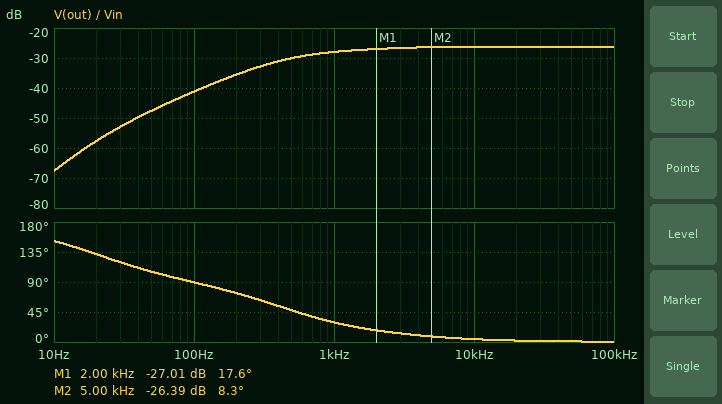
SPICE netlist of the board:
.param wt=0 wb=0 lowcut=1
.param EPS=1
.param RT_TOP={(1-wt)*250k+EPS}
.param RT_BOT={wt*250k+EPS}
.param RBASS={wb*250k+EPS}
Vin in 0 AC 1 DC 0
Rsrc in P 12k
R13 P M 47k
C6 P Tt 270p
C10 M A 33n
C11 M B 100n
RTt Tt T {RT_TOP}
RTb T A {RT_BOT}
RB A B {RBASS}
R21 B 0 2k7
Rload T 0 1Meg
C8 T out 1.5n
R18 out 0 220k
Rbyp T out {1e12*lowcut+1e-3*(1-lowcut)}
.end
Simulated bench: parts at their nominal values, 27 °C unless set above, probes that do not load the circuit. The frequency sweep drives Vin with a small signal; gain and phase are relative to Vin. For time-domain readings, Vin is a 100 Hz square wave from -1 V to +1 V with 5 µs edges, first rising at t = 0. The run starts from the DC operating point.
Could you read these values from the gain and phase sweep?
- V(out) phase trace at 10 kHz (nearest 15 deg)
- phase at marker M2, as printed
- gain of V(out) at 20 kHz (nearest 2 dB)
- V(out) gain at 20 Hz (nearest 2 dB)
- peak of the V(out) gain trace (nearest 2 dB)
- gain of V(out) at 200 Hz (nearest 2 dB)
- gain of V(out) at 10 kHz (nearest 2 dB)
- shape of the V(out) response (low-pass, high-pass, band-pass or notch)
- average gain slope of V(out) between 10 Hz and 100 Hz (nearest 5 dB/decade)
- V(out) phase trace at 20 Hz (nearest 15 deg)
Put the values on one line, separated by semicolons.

0 deg; 8.3 deg; -26 dB; -58 dB; -26 dB; -36 dB; -26 dB; high-pass; 25 dB/decade; 135 deg
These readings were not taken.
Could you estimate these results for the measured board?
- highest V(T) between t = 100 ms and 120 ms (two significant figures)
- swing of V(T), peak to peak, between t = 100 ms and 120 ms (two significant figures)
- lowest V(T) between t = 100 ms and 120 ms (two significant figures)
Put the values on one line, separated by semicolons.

67 mV; 130 mV; -67 mV
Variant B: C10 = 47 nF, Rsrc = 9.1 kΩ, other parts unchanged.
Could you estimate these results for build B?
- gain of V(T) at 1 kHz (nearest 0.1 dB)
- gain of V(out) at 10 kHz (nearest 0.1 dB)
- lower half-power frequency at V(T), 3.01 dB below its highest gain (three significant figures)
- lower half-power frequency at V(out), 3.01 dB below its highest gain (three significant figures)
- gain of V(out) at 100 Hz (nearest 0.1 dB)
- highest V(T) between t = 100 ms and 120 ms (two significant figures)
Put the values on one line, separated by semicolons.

-26.6 dB; -25.8 dB; 24.5 Hz; 635 Hz; -40.8 dB; 70 mV
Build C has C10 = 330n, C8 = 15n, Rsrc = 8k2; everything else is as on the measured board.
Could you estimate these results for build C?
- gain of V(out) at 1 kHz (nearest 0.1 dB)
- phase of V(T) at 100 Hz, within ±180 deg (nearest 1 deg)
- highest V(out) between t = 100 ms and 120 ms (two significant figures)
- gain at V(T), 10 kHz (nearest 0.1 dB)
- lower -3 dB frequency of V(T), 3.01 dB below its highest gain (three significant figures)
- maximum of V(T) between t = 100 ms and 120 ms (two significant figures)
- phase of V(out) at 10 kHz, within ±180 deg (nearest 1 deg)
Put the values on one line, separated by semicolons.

-26.5 dB; 4 deg; 92 mV; -25.6 dB; 8.58 Hz; 64 mV; 2 deg
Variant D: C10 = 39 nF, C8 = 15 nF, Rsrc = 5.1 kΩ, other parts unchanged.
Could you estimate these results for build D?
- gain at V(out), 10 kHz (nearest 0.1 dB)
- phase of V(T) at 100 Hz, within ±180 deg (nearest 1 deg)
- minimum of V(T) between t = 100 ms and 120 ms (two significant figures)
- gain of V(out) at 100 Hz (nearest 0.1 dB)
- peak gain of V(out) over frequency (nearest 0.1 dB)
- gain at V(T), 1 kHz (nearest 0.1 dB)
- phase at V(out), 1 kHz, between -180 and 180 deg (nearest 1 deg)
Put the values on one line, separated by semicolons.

-25.1 dB; 12 deg; -78 mV; -27.3 dB; -25.0 dB; -26.0 dB; 7 deg
